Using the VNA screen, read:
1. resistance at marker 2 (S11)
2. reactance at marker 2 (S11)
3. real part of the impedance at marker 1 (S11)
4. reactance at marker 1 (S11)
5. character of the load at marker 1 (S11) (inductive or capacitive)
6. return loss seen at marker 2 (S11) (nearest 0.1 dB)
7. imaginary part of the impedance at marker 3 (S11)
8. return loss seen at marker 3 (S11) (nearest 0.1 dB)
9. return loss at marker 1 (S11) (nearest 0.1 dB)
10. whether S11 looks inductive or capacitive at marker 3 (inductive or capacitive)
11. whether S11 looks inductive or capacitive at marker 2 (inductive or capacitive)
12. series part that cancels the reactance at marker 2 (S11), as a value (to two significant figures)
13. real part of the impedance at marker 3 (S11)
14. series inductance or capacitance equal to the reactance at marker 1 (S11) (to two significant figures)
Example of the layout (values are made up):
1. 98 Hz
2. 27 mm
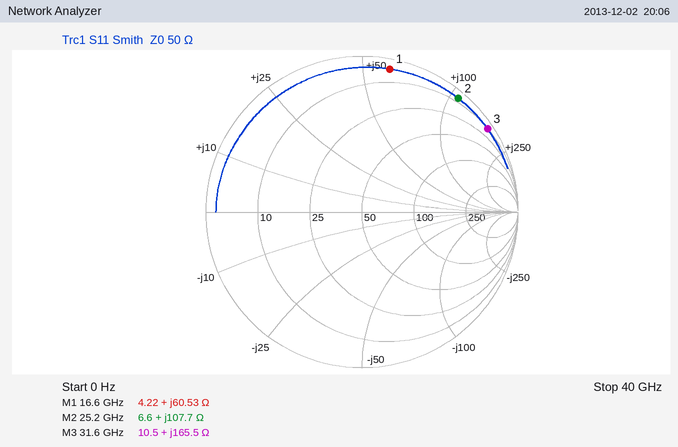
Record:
1. 6.6 Ω
2. +107.7 Ω
3. 4.22 Ω
4. +60.53 Ω
5. inductive
6. 0.4 dB
7. +165.5 Ω
8. 0.3 dB
9. 0.6 dB
10. inductive
11. inductive
12. 59 fF
13. 10.5 Ω
14. 580 pH
